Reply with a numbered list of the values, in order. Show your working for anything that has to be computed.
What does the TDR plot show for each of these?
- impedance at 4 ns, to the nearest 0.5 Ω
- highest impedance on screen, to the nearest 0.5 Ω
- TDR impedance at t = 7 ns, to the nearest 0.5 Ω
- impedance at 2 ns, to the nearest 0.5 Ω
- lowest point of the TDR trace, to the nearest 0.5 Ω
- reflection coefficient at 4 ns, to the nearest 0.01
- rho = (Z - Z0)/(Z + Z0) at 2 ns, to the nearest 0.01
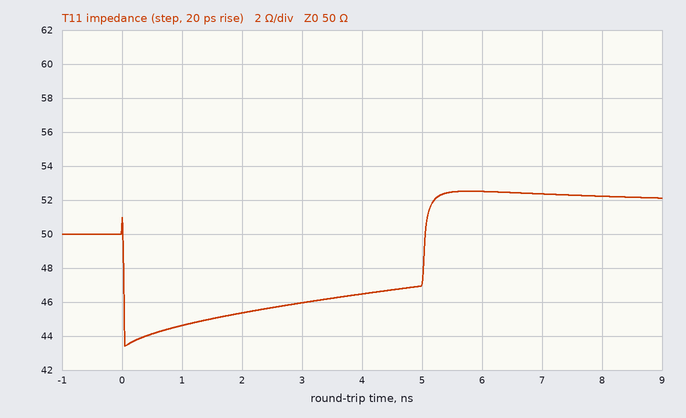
1. 46.5 Ω
2. 52.5 Ω
3. 52.5 Ω
4. 45.5 Ω
5. 43.5 Ω
6. (46.5 − 50)/(46.5 + 50) ≈ -0.04
7. (45.5 − 50)/(45.5 + 50) ≈ -0.05
